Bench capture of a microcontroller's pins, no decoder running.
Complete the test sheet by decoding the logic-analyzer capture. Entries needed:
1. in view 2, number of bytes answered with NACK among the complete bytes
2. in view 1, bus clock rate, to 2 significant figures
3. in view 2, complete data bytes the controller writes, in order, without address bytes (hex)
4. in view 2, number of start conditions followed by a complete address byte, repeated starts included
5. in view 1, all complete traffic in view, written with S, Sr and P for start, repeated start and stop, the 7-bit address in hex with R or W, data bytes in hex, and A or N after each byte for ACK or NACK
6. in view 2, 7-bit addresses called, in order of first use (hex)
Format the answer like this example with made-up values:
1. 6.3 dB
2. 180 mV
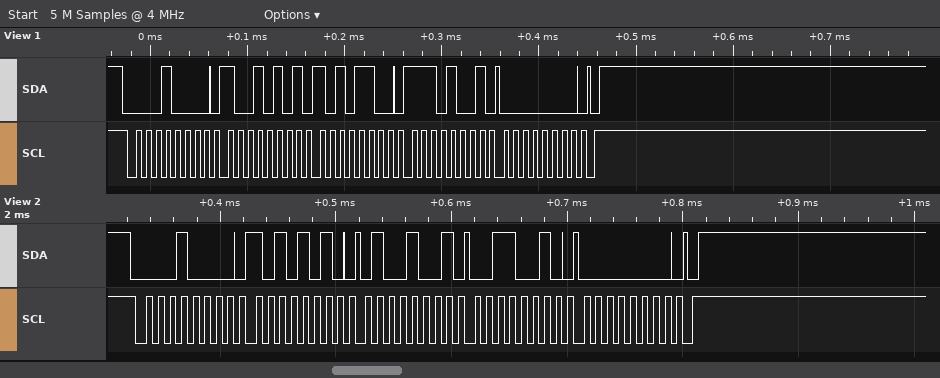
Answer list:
1. 0
2. 100 kHz
3. AA 49 32 00
4. 1
5. S 08W A 95 A AC A E9 A 00 A P
6. 0x08
